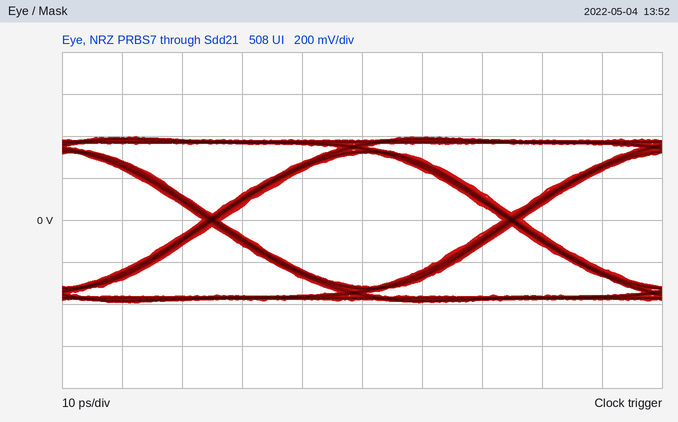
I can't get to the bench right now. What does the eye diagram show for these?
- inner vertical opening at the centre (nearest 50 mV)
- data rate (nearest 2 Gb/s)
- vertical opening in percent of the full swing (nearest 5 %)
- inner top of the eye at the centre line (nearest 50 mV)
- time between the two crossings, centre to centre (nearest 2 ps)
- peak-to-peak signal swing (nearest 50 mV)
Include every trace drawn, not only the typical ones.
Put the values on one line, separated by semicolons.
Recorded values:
650 mV; 20 Gb/s; 80 %; 300 mV; 50 ps; 800 mV
